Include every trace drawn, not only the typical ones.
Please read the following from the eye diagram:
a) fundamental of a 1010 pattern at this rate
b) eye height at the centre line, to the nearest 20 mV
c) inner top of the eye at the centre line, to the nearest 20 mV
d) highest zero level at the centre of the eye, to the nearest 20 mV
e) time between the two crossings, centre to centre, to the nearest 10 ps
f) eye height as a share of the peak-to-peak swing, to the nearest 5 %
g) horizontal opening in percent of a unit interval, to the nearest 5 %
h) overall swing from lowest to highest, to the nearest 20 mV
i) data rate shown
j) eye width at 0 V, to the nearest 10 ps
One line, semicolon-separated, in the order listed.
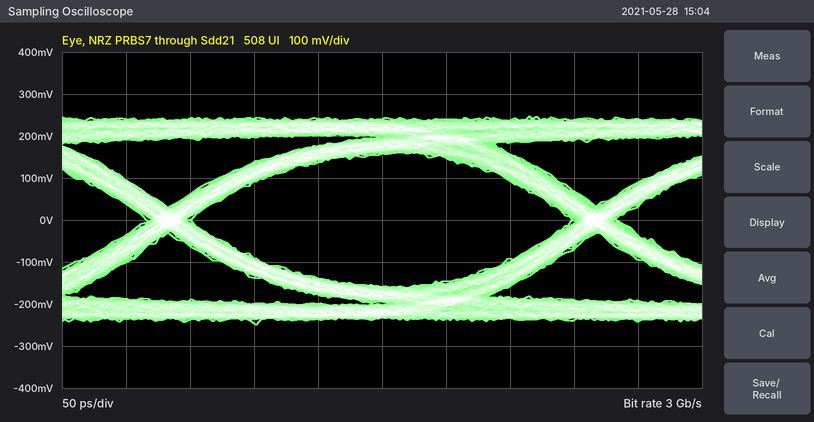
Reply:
1.5 GHz; 320 mV; 160 mV; -160 mV; 330 ps; 65 %; 90 %; 500 mV; 3 Gb/s; 300 ps
